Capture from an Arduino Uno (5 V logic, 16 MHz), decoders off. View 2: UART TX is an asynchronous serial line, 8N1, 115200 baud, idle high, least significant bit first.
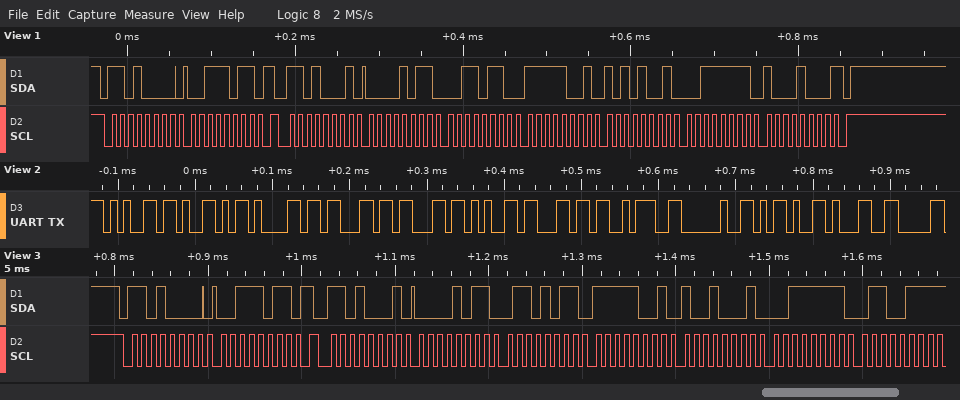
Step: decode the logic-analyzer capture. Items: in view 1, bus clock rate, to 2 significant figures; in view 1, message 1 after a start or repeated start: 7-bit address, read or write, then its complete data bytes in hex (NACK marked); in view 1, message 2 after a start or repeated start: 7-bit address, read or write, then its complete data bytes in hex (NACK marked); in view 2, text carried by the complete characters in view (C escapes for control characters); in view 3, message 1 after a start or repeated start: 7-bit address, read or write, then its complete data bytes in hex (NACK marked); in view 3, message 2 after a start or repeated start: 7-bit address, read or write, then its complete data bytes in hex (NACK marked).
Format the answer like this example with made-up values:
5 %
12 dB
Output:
100 kHz
0x68 write: 3B
0x68 read: 0B 36 F9 A9 3F 88 NACK
"eYaccel: -1"
0x68 write: 3B
0x68 read: 0B 6B F9 91 3F 67 NACK
